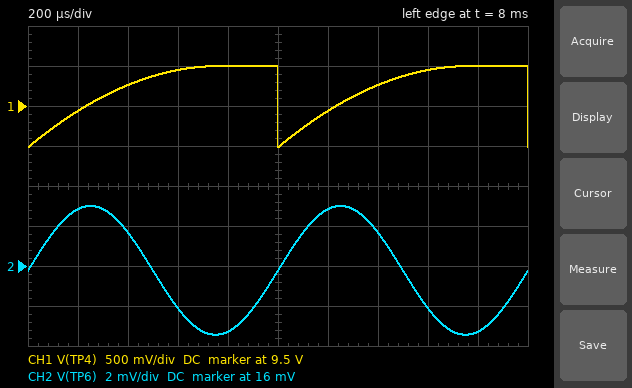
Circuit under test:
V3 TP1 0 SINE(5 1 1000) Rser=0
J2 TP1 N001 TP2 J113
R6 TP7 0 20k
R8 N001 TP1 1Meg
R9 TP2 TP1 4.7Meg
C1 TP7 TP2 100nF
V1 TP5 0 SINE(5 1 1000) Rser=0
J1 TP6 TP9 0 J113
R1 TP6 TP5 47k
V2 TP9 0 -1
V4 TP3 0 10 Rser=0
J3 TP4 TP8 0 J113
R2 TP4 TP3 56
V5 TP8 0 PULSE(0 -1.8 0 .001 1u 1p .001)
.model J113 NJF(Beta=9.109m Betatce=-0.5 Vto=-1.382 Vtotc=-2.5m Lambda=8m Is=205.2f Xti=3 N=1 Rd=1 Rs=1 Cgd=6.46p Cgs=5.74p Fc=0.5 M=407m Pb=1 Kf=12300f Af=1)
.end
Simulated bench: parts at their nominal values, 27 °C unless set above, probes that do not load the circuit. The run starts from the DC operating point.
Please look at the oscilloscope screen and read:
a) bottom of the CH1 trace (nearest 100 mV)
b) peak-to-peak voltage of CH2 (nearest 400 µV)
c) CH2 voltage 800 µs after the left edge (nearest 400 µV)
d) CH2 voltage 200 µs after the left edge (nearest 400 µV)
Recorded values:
9.0 V
6.4 mV
12.8 mV
18.8 mV
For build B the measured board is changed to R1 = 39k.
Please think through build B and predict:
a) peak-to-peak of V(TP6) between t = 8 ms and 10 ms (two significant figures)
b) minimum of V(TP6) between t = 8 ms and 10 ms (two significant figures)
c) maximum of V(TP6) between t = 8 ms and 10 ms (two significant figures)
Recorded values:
7.8 mV
15 mV
23 mV
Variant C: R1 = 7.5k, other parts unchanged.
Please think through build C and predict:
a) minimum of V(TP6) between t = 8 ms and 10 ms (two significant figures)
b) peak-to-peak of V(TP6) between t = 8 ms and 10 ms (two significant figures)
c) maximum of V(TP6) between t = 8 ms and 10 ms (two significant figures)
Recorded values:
85 mV
53 mV
140 mV
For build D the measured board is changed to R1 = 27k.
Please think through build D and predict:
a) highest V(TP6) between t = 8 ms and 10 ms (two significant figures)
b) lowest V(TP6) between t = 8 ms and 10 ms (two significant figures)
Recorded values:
34 mV
22 mV
